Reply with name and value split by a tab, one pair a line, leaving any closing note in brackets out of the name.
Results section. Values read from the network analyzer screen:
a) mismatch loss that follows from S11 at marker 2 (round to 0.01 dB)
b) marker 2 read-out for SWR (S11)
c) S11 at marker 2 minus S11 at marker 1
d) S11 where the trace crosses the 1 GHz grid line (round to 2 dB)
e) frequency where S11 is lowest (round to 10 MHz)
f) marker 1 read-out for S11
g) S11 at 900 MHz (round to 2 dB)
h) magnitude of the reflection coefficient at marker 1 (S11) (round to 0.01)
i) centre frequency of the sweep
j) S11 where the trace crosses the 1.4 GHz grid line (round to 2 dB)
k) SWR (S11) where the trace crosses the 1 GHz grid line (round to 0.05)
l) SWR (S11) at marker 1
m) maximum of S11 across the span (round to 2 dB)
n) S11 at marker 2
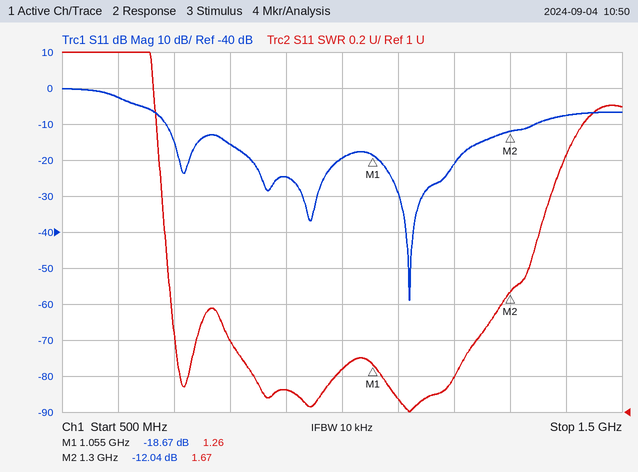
mismatch loss that follows from S11 at marker 2	0.28 dB
marker 2 read-out for SWR	1.67
S11 at marker 2 minus S11 at marker 1	6.63 dB
S11 where the trace crosses the 1 GHz grid line	-20 dB
frequency where S11 is lowest	1.12 GHz
marker 1 read-out for S11	-18.67 dB
S11 at 900 MHz	-24 dB
magnitude of the reflection coefficient at marker 1 (S11)	0.12
centre frequency of the sweep	1 GHz
S11 where the trace crosses the 1.4 GHz grid line	-8 dB
SWR (S11) where the trace crosses the 1 GHz grid line	1.25
SWR (S11) at marker 1	1.26
maximum of S11 across the span	0 dB
S11 at marker 2	-12.04 dB
